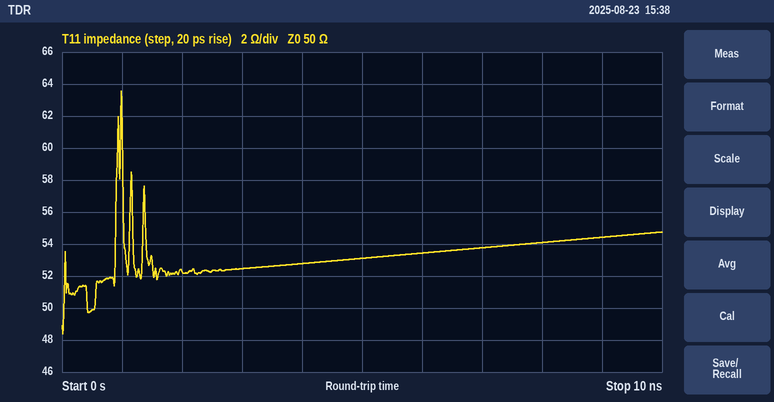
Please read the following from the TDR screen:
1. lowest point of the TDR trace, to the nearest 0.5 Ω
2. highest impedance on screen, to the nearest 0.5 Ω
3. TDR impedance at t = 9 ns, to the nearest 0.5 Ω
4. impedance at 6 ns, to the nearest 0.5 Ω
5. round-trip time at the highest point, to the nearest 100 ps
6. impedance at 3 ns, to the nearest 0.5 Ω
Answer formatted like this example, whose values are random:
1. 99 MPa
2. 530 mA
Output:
1. 48.5 Ω
2. 63.5 Ω
3. 54.5 Ω
4. 53.5 Ω
5. 1.0 ns
6. 52.5 Ω
